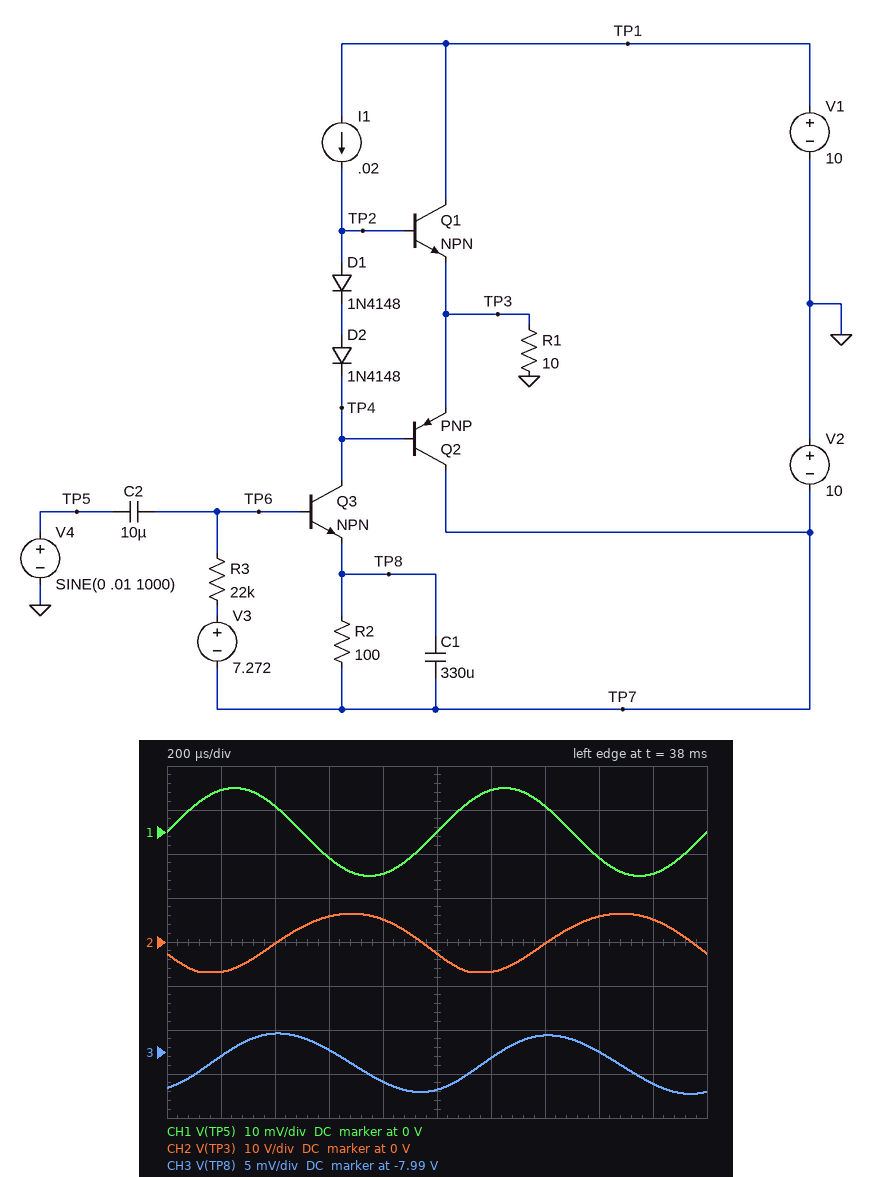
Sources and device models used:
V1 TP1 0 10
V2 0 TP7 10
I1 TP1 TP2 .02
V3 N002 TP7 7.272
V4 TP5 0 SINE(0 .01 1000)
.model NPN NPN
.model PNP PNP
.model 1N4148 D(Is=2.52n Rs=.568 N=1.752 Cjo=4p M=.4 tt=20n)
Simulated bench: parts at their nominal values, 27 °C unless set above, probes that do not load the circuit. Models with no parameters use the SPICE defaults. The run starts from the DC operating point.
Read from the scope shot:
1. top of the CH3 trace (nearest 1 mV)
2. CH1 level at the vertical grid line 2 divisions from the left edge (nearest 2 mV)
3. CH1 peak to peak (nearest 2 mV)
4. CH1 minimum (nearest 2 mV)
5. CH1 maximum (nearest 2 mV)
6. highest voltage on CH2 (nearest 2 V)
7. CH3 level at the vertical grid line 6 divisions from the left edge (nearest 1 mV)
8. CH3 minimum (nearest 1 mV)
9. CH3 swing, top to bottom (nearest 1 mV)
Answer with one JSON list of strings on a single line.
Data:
["-7.988 V", "6 mV", "20 mV", "-10 mV", "10 mV", "6 V", "-7.991 V", "-7.995 V", "7 mV"]
